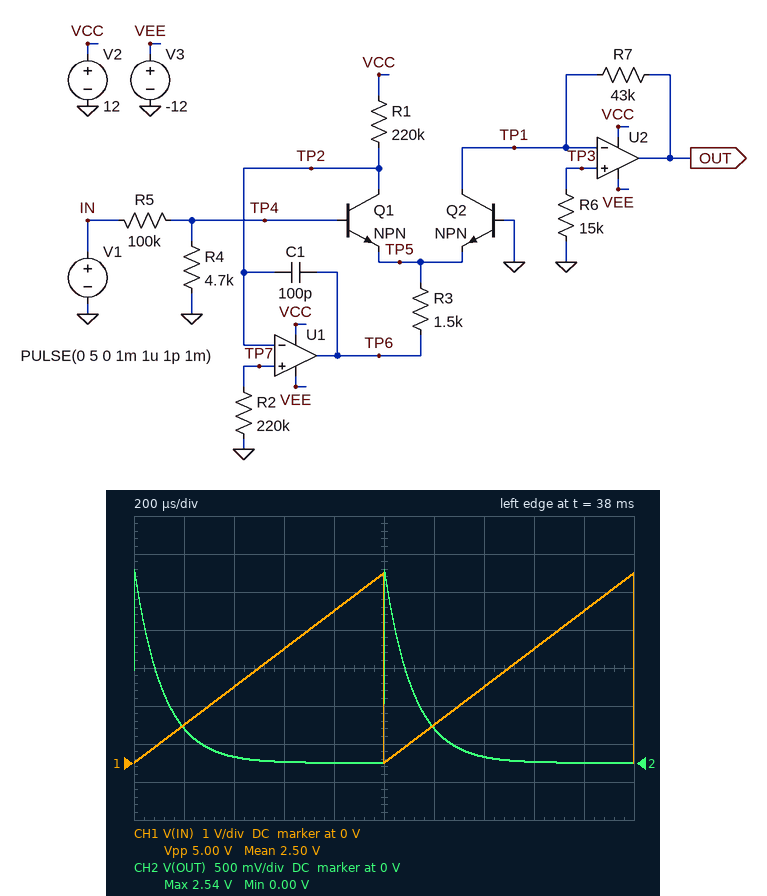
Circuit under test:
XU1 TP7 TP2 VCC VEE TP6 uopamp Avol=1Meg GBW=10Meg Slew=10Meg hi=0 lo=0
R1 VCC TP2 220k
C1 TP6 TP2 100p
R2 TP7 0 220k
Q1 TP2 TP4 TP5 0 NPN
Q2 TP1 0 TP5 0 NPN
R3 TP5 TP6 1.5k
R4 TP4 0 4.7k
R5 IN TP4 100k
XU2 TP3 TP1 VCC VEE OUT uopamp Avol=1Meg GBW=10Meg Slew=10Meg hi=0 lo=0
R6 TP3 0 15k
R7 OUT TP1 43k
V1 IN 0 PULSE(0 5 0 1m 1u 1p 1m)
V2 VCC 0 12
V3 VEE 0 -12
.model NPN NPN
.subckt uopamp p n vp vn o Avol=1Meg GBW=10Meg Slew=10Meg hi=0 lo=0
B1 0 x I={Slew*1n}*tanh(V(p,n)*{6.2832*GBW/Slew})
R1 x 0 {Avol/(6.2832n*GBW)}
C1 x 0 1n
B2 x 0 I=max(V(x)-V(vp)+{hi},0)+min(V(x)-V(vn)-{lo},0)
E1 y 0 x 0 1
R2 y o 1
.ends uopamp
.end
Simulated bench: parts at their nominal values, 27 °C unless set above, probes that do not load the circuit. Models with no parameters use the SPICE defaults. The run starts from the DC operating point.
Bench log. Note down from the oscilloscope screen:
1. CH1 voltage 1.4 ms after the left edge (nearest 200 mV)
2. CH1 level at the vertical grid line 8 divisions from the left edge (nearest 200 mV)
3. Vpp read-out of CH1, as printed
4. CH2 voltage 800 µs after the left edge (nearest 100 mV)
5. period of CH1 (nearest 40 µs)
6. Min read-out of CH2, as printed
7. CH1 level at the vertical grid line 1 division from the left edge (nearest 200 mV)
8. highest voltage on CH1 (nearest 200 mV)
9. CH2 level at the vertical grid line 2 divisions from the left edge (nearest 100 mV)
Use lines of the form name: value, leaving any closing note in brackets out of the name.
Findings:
CH1 voltage 1.4 ms after the left edge: 2.0 V
CH1 level at the vertical grid line 8 divisions from the left edge: 3.0 V
Vpp read-out of CH1, as printed: 5.00 V
CH2 voltage 800 µs after the left edge: 0 V
period of CH1: 1.00 ms
Min read-out of CH2, as printed: 0.00 V
CH1 level at the vertical grid line 1 division from the left edge: 1.0 V
highest voltage on CH1: 5.0 V
CH2 level at the vertical grid line 2 divisions from the left edge: 100 mV
